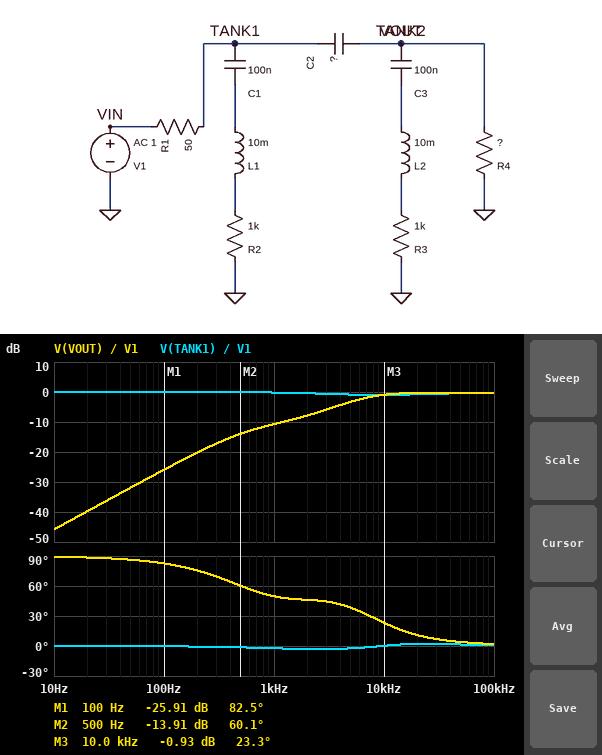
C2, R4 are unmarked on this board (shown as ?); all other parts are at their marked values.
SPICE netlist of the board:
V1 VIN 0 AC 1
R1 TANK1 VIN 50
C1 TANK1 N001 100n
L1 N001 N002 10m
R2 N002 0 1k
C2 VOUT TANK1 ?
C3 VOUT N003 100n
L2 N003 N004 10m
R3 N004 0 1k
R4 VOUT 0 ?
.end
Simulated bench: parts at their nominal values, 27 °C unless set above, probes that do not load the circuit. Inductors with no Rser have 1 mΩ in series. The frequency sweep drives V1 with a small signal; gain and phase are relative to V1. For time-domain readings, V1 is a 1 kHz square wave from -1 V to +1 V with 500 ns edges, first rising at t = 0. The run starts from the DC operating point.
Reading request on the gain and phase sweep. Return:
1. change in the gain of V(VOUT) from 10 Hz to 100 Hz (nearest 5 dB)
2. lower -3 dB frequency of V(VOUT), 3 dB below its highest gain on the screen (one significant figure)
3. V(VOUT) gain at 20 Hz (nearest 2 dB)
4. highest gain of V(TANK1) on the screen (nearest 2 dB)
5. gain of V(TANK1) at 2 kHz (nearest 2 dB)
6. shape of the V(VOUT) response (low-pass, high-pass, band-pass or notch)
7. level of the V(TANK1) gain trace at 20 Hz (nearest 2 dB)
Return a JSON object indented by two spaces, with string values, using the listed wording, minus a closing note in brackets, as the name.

{
  "change in the gain of V(VOUT) from 10 Hz to 100 Hz": "20 dB",
  "lower -3 dB frequency of V(VOUT), 3 dB below its highest gain on the screen": "5 kHz",
  "V(VOUT) gain at 20 Hz": "-40 dB",
  "highest gain of V(TANK1) on the screen": "0 dB",
  "gain of V(TANK1) at 2 kHz": "0 dB",
  "shape of the V(VOUT) response": "high-pass",
  "level of the V(TANK1) gain trace at 20 Hz": "0 dB"
}
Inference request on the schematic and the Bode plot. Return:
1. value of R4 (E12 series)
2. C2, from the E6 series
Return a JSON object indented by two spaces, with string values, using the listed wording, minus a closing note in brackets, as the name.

{
  "value of R4": "1.2 kΩ",
  "C2, from the E6 series": "68 nF"
}
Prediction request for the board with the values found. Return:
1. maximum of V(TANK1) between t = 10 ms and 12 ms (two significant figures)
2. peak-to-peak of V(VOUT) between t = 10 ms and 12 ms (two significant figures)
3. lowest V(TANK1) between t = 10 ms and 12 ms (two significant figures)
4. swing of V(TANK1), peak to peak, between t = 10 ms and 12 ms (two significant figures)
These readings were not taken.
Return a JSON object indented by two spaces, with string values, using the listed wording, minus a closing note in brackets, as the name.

{
  "maximum of V(TANK1) between t = 10 ms and 12 ms": "1.0 V",
  "peak-to-peak of V(VOUT) between t = 10 ms and 12 ms": "3.7 V",
  "lowest V(TANK1) between t = 10 ms and 12 ms": "-1.0 V",
  "swing of V(TANK1), peak to peak, between t = 10 ms and 12 ms": "2.0 V"
}
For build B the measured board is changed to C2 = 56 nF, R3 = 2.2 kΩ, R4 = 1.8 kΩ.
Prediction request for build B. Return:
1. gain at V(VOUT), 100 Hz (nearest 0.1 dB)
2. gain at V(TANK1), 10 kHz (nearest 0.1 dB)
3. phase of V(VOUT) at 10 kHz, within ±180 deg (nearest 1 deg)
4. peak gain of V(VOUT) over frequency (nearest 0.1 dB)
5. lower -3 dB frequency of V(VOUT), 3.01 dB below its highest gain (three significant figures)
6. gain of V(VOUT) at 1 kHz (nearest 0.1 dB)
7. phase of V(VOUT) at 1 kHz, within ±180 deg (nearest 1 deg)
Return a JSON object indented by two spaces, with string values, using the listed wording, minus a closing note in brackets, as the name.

{
  "gain at V(VOUT), 100 Hz": "-24.2 dB",
  "gain at V(TANK1), 10 kHz": "-0.7 dB",
  "phase of V(VOUT) at 10 kHz, within ±180 deg": "17 deg",
  "peak gain of V(VOUT) over frequency": "-0.2 dB",
  "lower -3 dB frequency of V(VOUT), 3.01 dB below its highest gain": "3.33 kHz",
  "gain of V(VOUT) at 1 kHz": "-9.5 dB",
  "phase of V(VOUT) at 1 kHz, within ±180 deg": "55 deg"
}
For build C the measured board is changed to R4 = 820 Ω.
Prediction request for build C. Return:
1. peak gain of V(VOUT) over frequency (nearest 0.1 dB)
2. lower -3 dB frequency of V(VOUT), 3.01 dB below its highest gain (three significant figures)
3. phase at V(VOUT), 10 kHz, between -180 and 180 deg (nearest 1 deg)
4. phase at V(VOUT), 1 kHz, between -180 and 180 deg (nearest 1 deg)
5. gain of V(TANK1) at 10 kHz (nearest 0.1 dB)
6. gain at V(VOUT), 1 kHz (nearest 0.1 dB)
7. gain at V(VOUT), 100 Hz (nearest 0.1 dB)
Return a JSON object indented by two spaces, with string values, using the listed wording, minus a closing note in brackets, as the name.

{
  "peak gain of V(VOUT) over frequency": "-0.5 dB",
  "lower -3 dB frequency of V(VOUT), 3.01 dB below its highest gain": "5.57 kHz",
  "phase at V(VOUT), 10 kHz, between -180 and 180 deg": "27 deg",
  "phase at V(VOUT), 1 kHz, between -180 and 180 deg": "57 deg",
  "gain of V(TANK1) at 10 kHz": "-1.1 dB",
  "gain at V(VOUT), 1 kHz": "-12.5 dB",
  "gain at V(VOUT), 100 Hz": "-29.2 dB"
}
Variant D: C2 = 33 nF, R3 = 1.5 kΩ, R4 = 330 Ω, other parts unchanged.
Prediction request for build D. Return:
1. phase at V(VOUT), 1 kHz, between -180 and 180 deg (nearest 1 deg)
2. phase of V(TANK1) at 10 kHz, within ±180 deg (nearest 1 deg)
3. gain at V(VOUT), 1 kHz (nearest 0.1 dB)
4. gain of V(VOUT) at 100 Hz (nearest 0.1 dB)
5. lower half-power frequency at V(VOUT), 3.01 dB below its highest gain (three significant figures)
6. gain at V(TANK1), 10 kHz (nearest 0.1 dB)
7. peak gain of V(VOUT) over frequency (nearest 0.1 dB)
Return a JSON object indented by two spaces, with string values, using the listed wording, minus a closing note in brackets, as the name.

{
  "phase at V(VOUT), 1 kHz, between -180 and 180 deg": "79 deg",
  "phase of V(TANK1) at 10 kHz, within ±180 deg": "-3 deg",
  "gain at V(VOUT), 1 kHz": "-24.4 dB",
  "gain of V(VOUT) at 100 Hz": "-43.3 dB",
  "lower half-power frequency at V(VOUT), 3.01 dB below its highest gain": "14.9 kHz",
  "gain at V(TANK1), 10 kHz": "-0.7 dB",
  "peak gain of V(VOUT) over frequency": "-1.2 dB"
}
